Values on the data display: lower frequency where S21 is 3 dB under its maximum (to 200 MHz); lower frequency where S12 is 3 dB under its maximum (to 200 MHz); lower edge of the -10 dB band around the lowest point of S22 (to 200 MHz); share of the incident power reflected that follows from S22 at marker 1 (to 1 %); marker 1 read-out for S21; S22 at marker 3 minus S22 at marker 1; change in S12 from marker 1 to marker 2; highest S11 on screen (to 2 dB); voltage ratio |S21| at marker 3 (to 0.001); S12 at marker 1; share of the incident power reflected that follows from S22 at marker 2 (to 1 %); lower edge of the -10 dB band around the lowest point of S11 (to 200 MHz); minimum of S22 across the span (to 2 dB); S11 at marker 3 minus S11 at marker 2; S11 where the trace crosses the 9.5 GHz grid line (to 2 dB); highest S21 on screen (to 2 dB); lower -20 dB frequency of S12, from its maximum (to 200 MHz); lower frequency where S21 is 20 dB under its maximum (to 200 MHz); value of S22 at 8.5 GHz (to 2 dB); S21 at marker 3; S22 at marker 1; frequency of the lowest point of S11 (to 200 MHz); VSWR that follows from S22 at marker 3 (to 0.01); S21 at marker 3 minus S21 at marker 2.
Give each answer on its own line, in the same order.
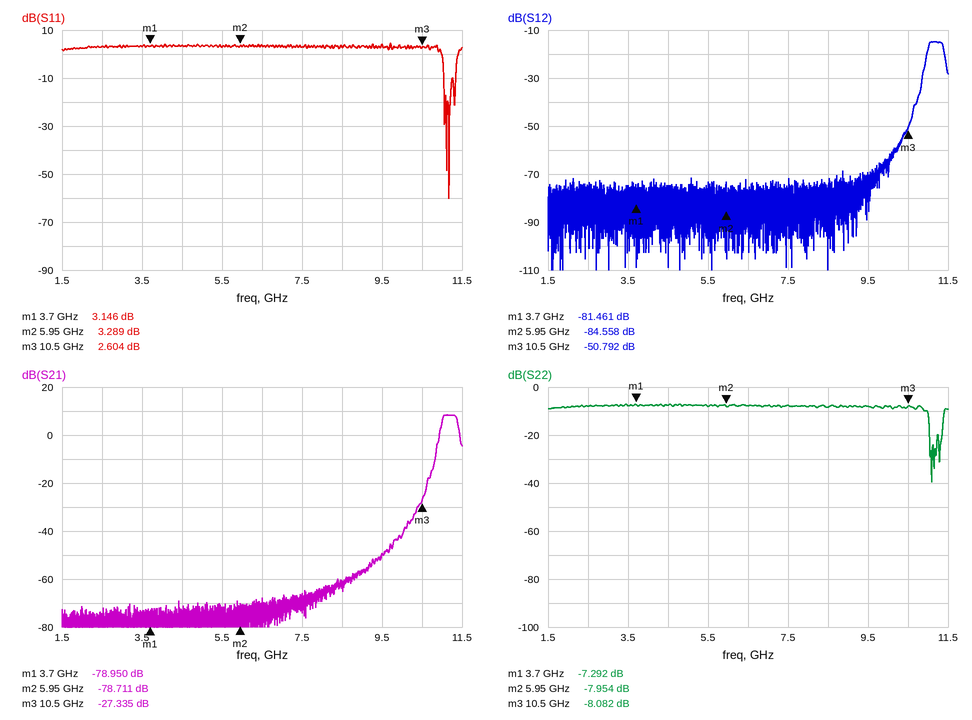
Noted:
11.0 GHz
11.0 GHz
11.0 GHz
19 %
-78.950 dB
-0.790 dB
-3.097 dB
4 dB
0.043
-81.461 dB
16 %
11.0 GHz
-40 dB
-0.685 dB
4 dB
8 dB
10.8 GHz
10.8 GHz
-8 dB
-27.335 dB
-7.292 dB
11.2 GHz
2.30
51.376 dB
